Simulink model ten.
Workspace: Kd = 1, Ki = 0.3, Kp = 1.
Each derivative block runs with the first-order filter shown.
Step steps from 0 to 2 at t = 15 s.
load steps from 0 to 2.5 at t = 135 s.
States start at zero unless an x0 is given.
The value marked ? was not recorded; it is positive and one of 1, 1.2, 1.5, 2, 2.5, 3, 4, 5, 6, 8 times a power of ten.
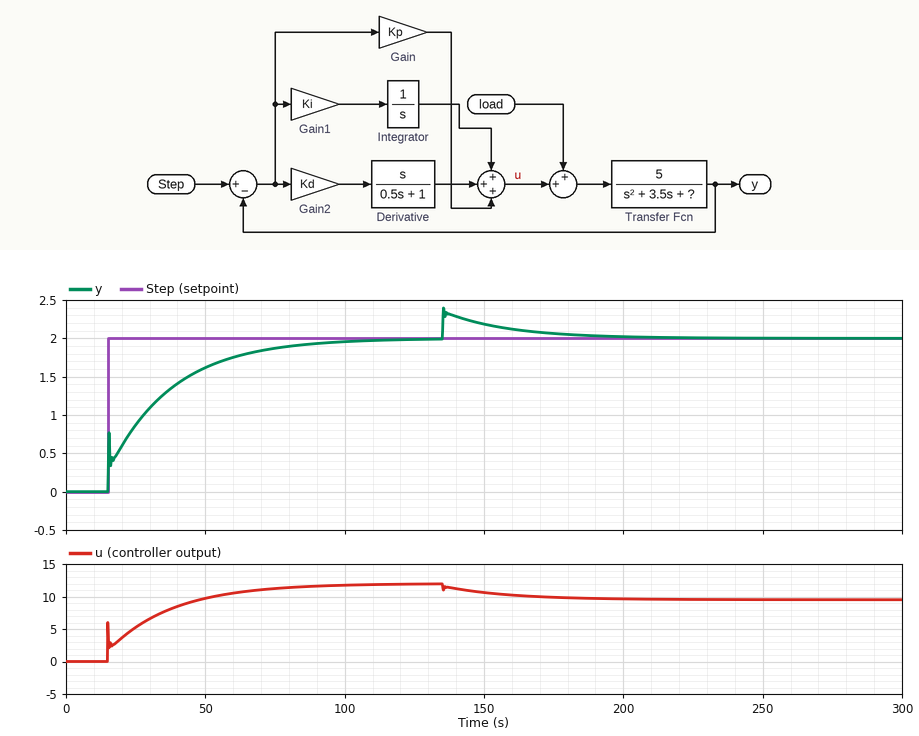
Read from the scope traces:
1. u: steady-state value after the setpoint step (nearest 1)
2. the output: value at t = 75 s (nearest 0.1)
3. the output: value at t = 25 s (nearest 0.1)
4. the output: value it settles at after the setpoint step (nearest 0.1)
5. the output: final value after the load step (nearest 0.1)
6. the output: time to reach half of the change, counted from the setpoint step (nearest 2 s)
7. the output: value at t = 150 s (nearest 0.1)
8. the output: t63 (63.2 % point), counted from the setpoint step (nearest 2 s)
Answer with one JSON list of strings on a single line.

["12", "1.9", "0.9", "2.0", "2.0", "12 s", "2.2", "20 s"]
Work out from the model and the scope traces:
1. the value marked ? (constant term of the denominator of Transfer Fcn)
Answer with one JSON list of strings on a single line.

["30"]
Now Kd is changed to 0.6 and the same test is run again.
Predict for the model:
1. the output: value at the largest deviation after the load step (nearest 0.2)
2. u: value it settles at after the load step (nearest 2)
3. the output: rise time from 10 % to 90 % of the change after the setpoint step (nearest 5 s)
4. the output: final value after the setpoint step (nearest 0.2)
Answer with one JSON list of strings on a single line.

["2.4", "10", "50 s", "2.0"]
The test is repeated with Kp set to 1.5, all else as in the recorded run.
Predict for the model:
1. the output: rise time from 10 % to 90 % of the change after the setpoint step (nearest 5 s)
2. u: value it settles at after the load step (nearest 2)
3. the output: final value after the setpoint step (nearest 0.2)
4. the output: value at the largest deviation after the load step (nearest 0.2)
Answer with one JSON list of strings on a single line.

["50 s", "10", "2.0", "2.4"]
